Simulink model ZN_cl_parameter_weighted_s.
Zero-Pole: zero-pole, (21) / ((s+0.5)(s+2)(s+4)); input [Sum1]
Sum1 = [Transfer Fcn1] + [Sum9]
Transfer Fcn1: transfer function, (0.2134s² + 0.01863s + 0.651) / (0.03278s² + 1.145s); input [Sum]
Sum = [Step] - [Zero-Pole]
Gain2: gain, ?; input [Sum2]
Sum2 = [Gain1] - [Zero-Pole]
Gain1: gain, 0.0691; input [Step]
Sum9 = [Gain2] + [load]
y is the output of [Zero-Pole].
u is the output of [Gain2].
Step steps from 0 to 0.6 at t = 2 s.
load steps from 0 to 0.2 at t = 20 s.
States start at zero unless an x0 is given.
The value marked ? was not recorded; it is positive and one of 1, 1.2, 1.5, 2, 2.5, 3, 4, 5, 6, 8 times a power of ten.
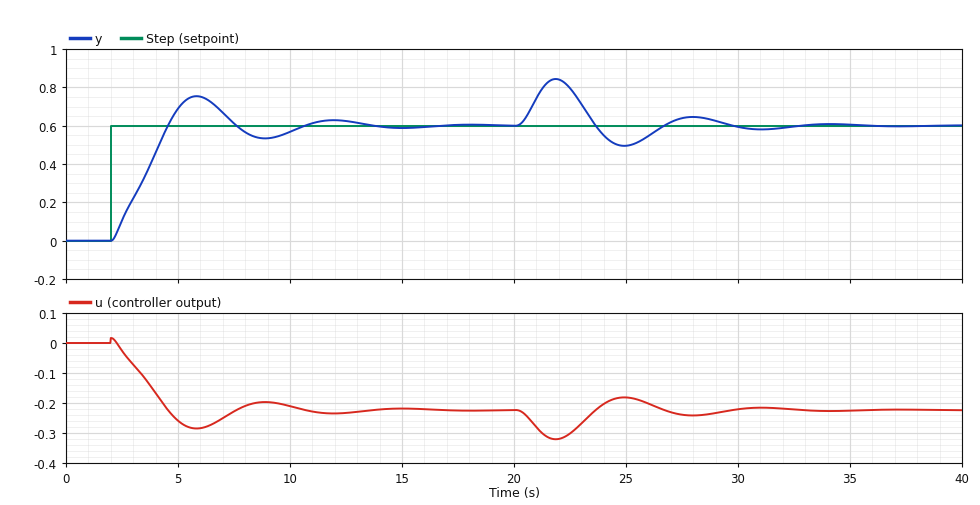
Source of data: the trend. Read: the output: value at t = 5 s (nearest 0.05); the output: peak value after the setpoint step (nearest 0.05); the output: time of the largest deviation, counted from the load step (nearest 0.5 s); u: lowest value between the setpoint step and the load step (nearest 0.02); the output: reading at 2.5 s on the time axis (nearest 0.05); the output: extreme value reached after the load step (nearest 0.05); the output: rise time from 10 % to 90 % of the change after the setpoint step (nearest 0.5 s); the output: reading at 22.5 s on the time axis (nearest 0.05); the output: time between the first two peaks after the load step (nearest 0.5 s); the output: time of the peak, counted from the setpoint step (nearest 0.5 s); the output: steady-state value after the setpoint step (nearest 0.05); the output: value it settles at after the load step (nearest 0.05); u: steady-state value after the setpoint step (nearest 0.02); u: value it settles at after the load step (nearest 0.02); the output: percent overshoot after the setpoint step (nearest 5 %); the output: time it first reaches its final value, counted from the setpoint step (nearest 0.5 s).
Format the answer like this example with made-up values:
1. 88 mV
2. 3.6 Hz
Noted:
1. 0.70
2. 0.75
3. 2.0 s
4. -0.28
5. 0.10
6. 0.85
7. 2.0 s
8. 0.80
9. 6.0 s
10. 4.0 s
11. 0.60
12. 0.60
13. -0.22
14. -0.22
15. 25 %
16. 2.5 s
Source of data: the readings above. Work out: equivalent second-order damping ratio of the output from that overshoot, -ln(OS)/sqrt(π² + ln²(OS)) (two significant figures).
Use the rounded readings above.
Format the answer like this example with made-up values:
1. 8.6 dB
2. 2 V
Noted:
1. 0.40
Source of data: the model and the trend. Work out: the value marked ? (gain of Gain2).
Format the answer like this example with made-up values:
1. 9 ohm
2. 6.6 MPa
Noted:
1. 0.4
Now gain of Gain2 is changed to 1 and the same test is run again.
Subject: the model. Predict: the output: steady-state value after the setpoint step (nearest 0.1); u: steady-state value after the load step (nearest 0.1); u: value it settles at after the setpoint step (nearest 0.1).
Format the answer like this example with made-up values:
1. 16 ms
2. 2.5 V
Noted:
1. 0.6
2. -0.6
3. -0.6
